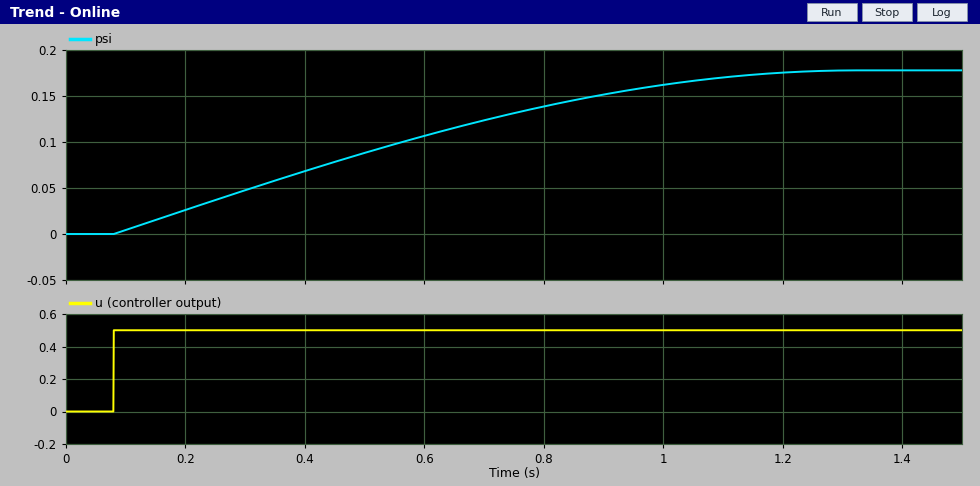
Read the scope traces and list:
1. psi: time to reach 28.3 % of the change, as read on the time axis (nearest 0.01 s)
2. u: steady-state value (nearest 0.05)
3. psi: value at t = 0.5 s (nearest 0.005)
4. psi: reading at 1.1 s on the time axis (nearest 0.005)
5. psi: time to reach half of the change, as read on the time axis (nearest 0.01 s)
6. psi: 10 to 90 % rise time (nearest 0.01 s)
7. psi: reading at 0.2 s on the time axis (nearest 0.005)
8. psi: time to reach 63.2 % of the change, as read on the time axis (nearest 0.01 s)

0.31 s
0.50
0.090
0.170
0.50 s
0.82 s
0.025
0.63 s
